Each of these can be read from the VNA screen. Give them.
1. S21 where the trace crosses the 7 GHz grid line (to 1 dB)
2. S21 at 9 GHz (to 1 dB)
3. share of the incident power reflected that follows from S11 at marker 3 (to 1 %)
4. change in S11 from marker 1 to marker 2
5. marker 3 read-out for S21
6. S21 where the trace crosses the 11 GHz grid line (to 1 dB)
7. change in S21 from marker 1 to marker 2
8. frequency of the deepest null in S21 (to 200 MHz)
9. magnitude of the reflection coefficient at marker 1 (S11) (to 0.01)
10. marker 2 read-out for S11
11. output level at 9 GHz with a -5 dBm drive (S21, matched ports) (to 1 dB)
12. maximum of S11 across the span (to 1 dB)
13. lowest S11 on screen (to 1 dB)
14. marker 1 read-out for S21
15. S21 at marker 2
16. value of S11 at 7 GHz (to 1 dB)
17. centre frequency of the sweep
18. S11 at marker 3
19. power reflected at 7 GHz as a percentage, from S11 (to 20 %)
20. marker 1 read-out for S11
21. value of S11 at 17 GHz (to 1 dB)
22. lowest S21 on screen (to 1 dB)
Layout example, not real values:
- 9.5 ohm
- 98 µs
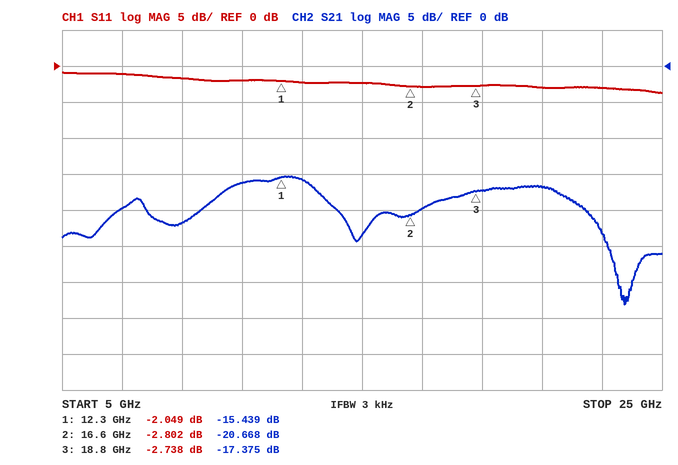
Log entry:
- -20 dB
- -22 dB
- 53 %
- -0.753 dB
- -17.375 dB
- -16 dB
- -5.229 dB
- 23.8 GHz
- 0.79
- -2.802 dB
- -27 dBm
- -1 dB
- -4 dB
- -15.439 dB
- -20.668 dB
- -1 dB
- 15 GHz
- -2.738 dB
- 80 %
- -2.049 dB
- -3 dB
- -33 dB
